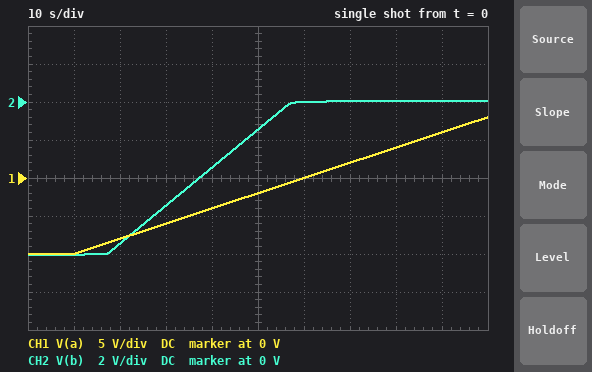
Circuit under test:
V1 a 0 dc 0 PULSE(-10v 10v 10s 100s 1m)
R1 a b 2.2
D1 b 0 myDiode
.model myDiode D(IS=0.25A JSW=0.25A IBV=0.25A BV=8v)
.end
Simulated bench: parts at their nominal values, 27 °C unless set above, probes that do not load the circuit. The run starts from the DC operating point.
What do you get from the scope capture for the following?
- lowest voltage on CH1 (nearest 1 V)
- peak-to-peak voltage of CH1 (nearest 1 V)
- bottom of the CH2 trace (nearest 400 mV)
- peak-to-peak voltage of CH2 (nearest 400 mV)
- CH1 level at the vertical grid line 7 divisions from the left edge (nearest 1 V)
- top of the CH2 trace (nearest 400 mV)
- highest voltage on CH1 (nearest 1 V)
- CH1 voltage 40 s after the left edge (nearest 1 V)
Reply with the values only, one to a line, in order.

-10 V
18 V
-8.0 V
8.0 V
2 V
0 V
8 V
-4 V
